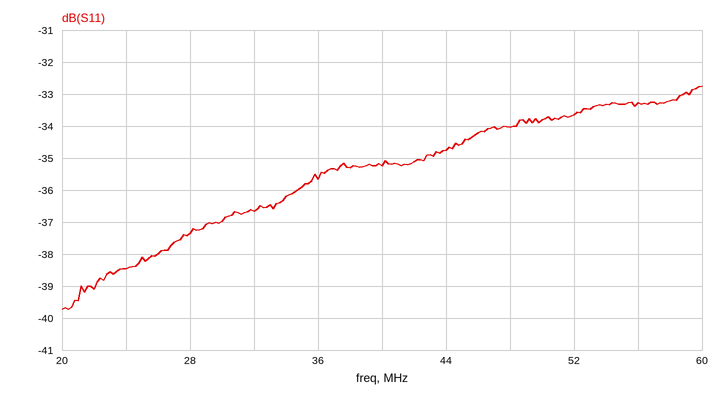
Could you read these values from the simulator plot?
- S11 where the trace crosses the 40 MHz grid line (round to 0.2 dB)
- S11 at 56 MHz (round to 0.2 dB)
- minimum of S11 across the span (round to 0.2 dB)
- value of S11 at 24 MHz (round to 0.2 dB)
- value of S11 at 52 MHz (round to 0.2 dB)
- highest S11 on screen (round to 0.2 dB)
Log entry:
-35.2 dB
-33.2 dB
-39.8 dB
-38.4 dB
-33.6 dB
-32.8 dB
